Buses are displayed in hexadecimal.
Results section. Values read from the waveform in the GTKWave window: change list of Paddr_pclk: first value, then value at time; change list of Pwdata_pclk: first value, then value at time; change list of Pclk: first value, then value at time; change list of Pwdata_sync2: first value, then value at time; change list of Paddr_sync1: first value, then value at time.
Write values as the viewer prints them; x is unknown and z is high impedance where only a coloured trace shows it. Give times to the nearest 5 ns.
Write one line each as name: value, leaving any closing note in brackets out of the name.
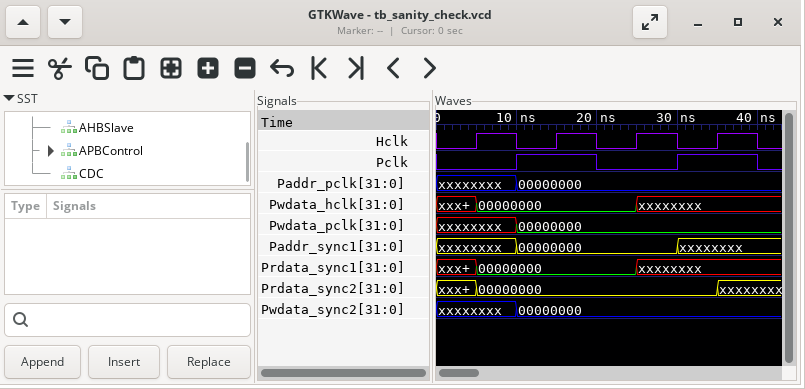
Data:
change list of Paddr_pclk: first value, then value at time: xxxxxxxx, 00000000 at 10 ns
change list of Pwdata_pclk: first value, then value at time: xxxxxxxx, 00000000 at 10 ns
change list of Pclk: first value, then value at time: 0, 1 at 10 ns, 0 at 20 ns, 1 at 30 ns, 0 at 40 ns
change list of Pwdata_sync2: first value, then value at time: xxxxxxxx, 00000000 at 10 ns
change list of Paddr_sync1: first value, then value at time: xxxxxxxx, 00000000 at 10 ns, xxxxxxxx at 30 ns
